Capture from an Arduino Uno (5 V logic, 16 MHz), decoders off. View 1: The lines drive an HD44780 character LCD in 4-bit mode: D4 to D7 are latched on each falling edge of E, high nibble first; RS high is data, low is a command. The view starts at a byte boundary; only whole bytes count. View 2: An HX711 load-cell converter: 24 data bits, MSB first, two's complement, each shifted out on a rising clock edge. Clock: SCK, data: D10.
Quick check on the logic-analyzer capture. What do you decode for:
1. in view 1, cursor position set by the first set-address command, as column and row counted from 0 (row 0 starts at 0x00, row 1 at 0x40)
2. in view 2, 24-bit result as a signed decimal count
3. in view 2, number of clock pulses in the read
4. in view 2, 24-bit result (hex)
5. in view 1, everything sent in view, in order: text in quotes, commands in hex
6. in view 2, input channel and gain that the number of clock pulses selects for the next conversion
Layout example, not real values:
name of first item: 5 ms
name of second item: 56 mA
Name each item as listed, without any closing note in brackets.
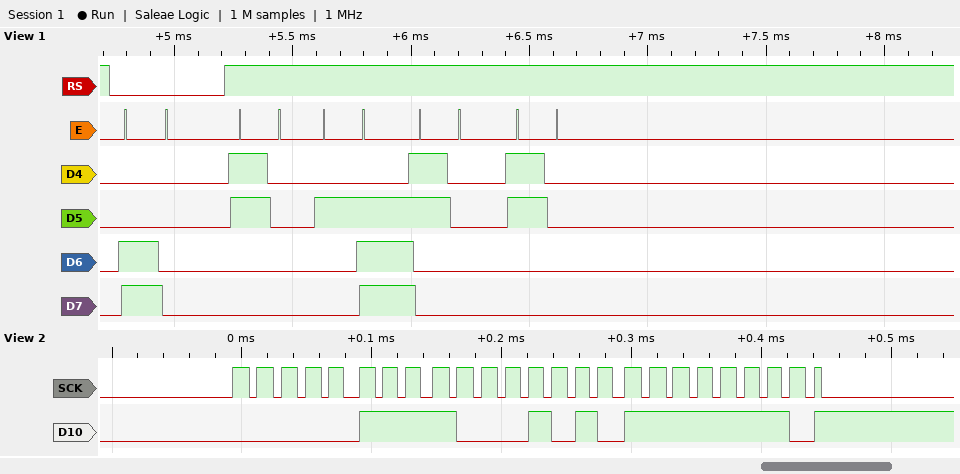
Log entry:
in view 1, cursor position set by the first set-address command, as column and row counted from 0: column 0, row 1
in view 2, 24-bit result as a signed decimal count: 494334
in view 2, number of clock pulses in the read: 25
in view 2, 24-bit result: 0x078AFE
in view 1, everything sent in view, in order: text in quotes, commands in hex: 0xC0 "0.00"
in view 2, input channel and gain that the number of clock pulses selects for the next conversion: channel A, gain 128
